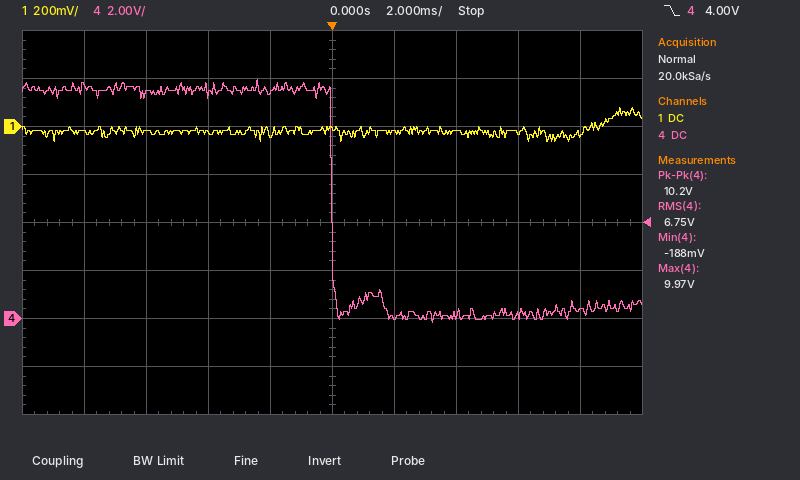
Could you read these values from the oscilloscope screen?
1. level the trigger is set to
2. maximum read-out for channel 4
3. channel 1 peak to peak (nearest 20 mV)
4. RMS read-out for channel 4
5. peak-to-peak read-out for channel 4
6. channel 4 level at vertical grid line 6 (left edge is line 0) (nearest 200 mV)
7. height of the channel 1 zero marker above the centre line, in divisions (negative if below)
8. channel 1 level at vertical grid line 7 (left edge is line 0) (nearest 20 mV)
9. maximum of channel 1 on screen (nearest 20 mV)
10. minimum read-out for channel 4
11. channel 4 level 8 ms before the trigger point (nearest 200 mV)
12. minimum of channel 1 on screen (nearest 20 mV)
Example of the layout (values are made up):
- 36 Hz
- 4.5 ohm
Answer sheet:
- 4.00 V
- 9.97 V
- 140 mV
- 6.75 V
- 10.2 V
- 0.0 V
- +2.0 div
- -20 mV
- 80 mV
- -188 mV
- 9.6 V
- -60 mV
